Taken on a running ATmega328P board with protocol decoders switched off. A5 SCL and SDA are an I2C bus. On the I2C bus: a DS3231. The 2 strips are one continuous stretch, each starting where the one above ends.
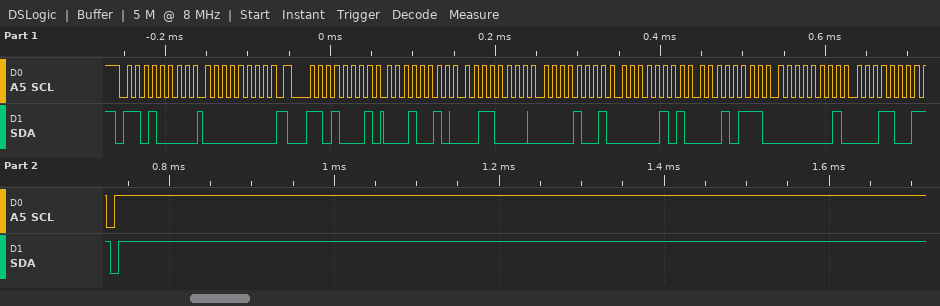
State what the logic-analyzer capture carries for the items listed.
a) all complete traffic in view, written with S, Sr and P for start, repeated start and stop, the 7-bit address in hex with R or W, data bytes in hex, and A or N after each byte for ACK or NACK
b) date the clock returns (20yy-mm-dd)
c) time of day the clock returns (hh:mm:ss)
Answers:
S 68W A 00 A Sr 68R A 12 A 30 A 09 A 05 A 17 A 01 A 19 N P
2019-01-17
09:30:12
